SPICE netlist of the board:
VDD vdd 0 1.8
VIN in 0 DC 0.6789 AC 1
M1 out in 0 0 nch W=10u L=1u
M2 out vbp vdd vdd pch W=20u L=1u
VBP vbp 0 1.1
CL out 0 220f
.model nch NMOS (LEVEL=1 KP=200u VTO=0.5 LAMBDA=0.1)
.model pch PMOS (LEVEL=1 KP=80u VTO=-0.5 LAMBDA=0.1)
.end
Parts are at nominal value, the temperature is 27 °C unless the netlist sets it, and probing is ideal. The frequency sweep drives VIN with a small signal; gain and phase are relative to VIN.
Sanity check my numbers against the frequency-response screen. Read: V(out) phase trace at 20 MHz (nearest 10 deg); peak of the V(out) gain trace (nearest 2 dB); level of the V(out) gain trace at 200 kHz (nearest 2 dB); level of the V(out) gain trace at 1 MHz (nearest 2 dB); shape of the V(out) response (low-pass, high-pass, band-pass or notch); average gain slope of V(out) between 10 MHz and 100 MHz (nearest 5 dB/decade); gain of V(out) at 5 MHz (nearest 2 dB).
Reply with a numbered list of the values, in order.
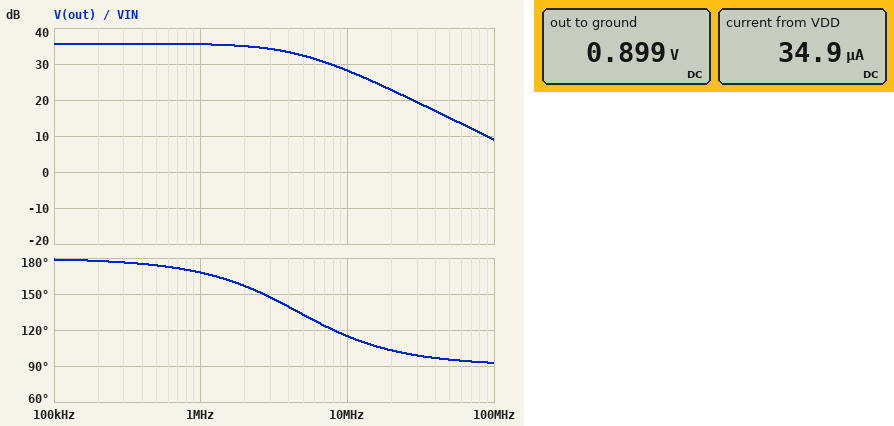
1. 100 deg
2. 36 dB
3. 36 dB
4. 36 dB
5. low-pass
6. -20 dB/decade
7. 32 dB
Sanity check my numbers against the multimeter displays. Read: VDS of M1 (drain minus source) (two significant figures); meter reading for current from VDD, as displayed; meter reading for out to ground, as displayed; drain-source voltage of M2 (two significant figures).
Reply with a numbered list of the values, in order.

1. 900 mV
2. 34.9 µA
3. 0.899 V
4. -900 mV
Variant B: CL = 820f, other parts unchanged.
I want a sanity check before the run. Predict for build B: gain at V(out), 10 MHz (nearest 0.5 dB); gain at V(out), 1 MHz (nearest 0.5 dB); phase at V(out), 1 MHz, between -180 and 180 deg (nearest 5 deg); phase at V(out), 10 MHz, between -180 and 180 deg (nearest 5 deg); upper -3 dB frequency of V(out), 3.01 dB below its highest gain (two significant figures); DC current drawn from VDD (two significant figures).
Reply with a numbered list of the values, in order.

1. 17.5 dB
2. 33.5 dB
3. 140 deg
4. 95 deg
5. 1.2 MHz
6. 35 µA
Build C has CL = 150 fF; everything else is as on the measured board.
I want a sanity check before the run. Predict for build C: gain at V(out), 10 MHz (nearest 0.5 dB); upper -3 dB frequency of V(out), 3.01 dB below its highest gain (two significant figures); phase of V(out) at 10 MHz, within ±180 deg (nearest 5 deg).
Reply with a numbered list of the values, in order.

1. 30.5 dB
2. 6.8 MHz
3. 125 deg
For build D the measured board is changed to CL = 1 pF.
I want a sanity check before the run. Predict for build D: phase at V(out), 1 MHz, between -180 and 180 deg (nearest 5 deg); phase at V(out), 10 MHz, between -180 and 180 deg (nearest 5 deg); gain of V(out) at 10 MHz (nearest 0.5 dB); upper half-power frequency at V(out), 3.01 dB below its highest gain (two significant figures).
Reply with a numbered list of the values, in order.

1. 135 deg
2. 95 deg
3. 16.0 dB
4. 1.0 MHz
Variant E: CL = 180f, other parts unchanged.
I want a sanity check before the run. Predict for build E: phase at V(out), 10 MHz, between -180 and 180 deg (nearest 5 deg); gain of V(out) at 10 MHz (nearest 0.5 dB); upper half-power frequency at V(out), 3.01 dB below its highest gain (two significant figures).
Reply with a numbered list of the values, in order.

1. 120 deg
2. 29.5 dB
3. 5.7 MHz
